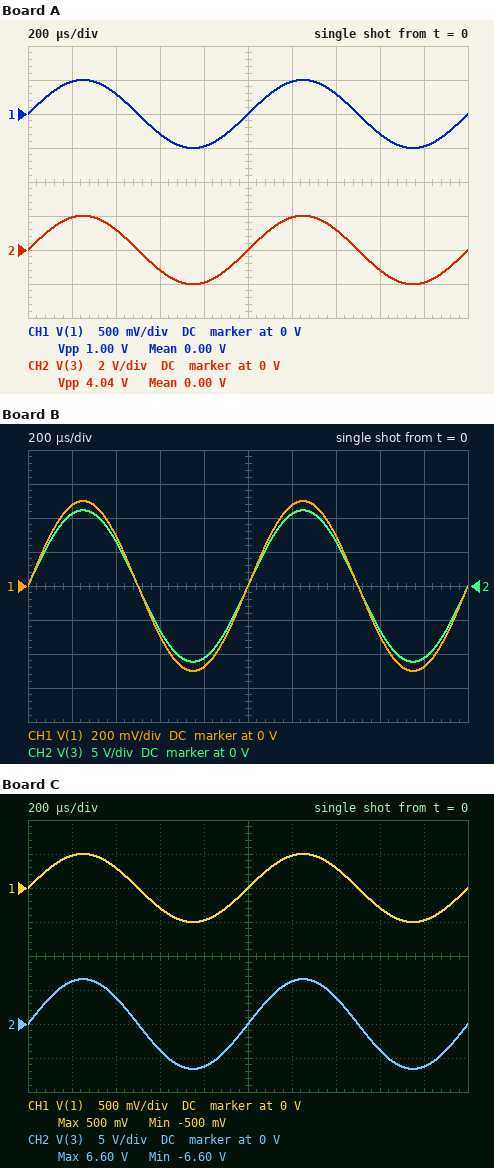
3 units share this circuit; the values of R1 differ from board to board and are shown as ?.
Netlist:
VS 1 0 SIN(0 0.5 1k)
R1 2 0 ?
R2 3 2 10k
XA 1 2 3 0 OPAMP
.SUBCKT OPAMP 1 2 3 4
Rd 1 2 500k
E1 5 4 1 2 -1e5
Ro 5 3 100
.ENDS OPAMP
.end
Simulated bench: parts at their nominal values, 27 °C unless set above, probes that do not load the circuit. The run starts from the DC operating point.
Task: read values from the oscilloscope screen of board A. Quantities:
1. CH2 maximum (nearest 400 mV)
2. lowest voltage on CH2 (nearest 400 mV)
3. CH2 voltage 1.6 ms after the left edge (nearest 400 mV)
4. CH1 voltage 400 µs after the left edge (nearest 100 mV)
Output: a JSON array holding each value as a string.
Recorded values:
["2.0 V", "-2.0 V", "-1.2 V", "300 mV"]
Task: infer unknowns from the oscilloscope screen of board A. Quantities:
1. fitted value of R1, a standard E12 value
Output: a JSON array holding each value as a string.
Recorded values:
["3.3 kΩ"]
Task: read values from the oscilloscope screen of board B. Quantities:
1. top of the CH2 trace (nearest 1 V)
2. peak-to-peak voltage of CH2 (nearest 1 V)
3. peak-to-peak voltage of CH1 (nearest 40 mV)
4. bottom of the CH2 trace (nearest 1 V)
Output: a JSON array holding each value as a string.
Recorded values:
["11 V", "22 V", "1.00 V", "-11 V"]
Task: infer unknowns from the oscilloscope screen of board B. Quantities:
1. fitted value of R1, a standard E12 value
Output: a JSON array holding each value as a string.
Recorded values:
["470 Ω"]
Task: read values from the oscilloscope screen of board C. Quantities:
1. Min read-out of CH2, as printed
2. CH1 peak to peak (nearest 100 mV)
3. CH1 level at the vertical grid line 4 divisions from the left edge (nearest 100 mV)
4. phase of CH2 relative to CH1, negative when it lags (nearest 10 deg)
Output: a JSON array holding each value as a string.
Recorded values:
["-6.60 V", "1.0 V", "-500 mV", "0 deg"]
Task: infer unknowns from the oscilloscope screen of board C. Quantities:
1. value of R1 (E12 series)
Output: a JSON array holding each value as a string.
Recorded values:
["820 Ω"]
